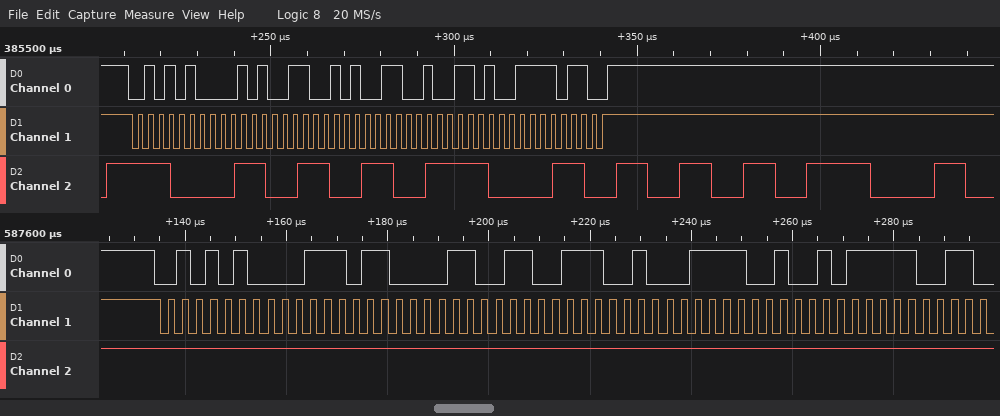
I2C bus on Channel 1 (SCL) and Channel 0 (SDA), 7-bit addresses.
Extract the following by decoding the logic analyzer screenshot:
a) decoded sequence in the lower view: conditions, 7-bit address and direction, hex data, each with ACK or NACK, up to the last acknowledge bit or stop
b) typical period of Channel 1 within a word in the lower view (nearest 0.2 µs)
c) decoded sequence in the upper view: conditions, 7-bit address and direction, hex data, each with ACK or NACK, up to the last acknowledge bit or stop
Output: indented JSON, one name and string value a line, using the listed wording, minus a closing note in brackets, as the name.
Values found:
{
  "decoded sequence in the lower view: conditions, 7-bit address and direction, hex data, each with ACK or NACK, up to the last acknowledge bit or stop": "start, address 2A write ACK, 76 ACK, 33 ACK, 72 ACK, 79 ACK, 5F ACK",
  "typical period of Channel 1 within a word in the lower view": "2.8 µs",
  "decoded sequence in the upper view: conditions, 7-bit address and direction, hex data, each with ACK or NACK, up to the last acknowledge bit or stop": "start, address 2A write ACK, 53 ACK, 53 ACK, 4D ACK, 7B ACK, stop"
}
